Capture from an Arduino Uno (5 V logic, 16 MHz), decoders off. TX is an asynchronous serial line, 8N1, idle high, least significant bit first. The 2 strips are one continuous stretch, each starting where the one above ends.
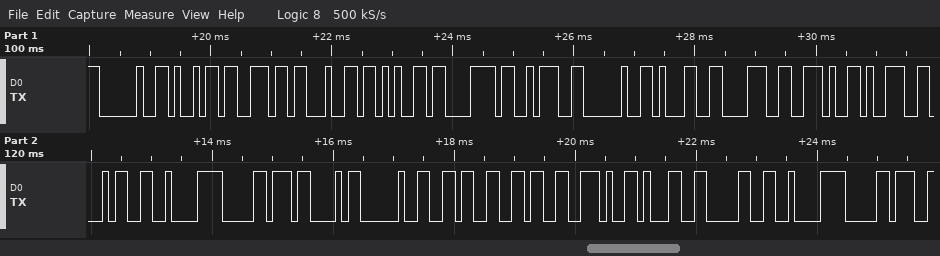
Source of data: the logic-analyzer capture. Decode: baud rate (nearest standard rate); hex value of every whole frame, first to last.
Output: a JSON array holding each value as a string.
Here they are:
["9600 baud", "20 69 6E 64 65 78 3A 20 31 38 2E 39 34 C2 B0 43 20 36 36 2E 31 30 C2 B0"]
